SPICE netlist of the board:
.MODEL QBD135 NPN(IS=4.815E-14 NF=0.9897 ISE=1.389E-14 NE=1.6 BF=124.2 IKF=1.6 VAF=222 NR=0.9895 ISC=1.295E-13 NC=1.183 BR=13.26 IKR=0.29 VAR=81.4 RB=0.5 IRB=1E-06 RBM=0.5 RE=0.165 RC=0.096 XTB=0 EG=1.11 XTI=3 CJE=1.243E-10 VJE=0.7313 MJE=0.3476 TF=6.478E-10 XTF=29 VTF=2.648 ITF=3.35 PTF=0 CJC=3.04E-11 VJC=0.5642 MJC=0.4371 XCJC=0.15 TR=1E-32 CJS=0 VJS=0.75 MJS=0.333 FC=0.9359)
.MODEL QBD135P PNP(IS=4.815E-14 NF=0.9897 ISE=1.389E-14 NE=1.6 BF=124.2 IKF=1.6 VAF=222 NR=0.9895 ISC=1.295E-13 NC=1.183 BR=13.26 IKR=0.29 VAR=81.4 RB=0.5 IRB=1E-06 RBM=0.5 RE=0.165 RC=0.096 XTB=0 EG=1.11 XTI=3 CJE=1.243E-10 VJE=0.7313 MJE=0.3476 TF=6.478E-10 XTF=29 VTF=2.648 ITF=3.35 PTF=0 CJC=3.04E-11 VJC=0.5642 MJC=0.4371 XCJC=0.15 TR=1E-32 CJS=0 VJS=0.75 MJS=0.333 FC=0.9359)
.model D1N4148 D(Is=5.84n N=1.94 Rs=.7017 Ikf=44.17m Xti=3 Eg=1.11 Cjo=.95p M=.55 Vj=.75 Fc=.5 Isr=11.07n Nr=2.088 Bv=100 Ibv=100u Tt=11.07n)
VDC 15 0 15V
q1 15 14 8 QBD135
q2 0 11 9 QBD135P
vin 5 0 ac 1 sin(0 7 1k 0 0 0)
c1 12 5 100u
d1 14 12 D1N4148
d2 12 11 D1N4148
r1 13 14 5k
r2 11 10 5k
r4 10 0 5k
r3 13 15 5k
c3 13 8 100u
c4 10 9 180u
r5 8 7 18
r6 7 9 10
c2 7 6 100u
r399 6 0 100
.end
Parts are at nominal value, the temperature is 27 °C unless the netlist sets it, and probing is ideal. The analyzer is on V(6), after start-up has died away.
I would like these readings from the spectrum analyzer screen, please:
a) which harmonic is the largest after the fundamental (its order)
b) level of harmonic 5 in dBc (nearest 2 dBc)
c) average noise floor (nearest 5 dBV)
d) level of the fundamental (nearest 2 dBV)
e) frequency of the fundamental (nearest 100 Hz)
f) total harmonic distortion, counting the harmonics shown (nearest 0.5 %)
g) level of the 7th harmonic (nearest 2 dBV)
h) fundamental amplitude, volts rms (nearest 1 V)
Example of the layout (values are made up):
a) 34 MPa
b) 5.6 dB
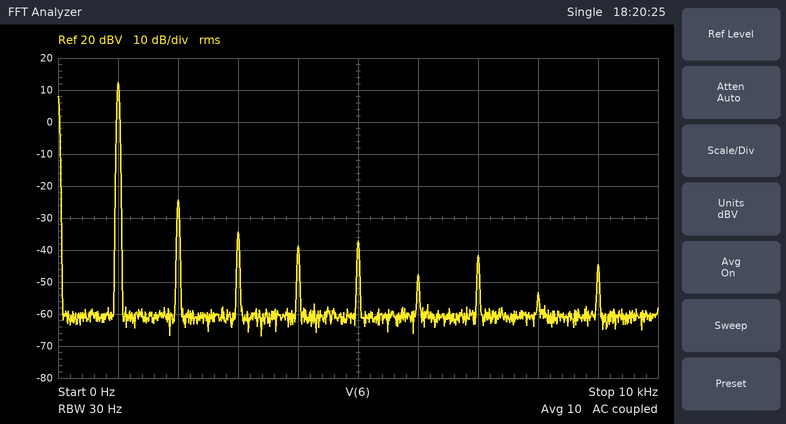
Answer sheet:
a) 2
b) -50 dBc
c) -60 dBV
d) 12 dBV
e) 1.0 kHz
f) 1.5 %
g) -42 dBV
h) 4 V
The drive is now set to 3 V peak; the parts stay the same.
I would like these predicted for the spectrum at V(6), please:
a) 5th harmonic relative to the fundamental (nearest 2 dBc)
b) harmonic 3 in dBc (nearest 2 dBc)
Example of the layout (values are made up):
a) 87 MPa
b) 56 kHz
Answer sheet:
a) -46 dBc
b) -40 dBc
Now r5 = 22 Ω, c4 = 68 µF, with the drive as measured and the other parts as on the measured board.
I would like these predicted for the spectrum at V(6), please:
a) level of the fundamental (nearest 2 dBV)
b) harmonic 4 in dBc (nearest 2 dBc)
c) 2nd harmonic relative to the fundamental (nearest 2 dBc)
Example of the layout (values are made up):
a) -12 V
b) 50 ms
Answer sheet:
a) 12 dBV
b) -48 dBc
c) -34 dBc
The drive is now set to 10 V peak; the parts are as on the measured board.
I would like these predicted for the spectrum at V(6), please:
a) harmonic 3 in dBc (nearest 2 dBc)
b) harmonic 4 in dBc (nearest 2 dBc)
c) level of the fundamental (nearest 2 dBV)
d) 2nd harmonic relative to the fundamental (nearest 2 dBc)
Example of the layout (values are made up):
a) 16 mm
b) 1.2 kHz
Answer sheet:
a) -20 dBc
b) -44 dBc
c) 14 dBV
d) -40 dBc
